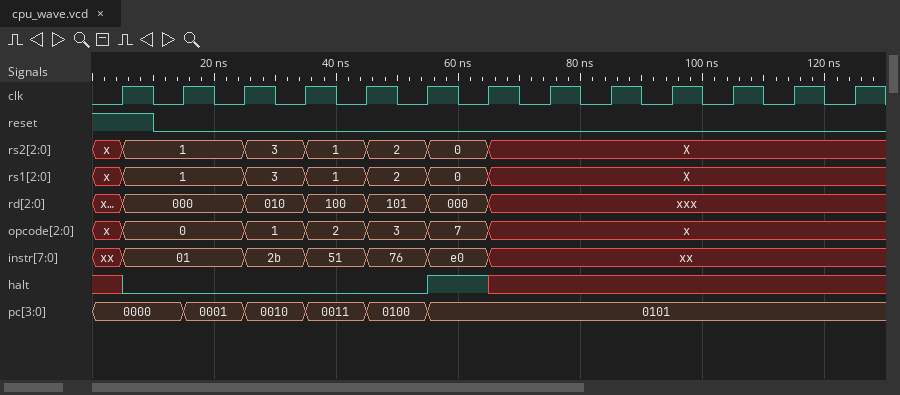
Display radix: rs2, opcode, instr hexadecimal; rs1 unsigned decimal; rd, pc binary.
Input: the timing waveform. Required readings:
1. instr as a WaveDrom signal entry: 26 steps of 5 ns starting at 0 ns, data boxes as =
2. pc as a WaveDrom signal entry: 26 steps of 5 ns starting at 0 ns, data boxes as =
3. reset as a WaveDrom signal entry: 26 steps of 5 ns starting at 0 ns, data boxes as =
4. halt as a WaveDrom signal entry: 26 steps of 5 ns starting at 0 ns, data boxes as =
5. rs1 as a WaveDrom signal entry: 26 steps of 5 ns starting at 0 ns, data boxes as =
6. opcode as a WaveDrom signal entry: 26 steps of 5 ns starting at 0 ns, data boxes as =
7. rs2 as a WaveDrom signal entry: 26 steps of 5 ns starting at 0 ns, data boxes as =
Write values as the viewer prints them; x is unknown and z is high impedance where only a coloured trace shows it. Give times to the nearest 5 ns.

{name: 'instr', wave: 'x=...=.=.=.=.x............', data: '01 2b 51 76 e0'}
{name: 'pc', wave: '=..=.=.=.=.=..............', data: '0000 0001 0010 0011 0100 0101'}
{name: 'reset', wave: '1.0.......................'}
{name: 'halt', wave: 'x0.........1.x............'}
{name: 'rs1', wave: 'x=...=.=.=.=.=............', data: '1 3 1 2 0 X'}
{name: 'opcode', wave: 'x=...=.=.=.=.x............', data: '0 1 2 3 7'}
{name: 'rs2', wave: 'x=...=.=.=.=.=............', data: '1 3 1 2 0 X'}
